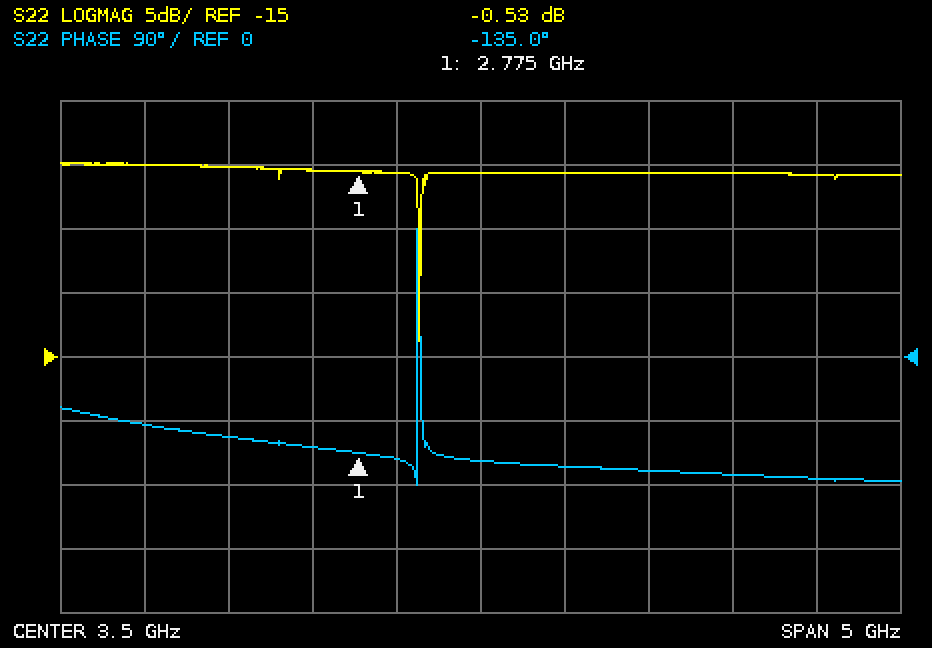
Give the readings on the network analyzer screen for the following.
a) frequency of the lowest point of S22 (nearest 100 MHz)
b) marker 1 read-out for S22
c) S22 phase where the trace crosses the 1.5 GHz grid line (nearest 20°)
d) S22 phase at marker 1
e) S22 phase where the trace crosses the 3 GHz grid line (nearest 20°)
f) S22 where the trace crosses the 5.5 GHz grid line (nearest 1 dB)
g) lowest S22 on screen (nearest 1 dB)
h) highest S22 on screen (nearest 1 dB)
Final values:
3.1 GHz
-0.53 dB
-100°
-135.0°
-140°
-1 dB
-14 dB
0 dB
